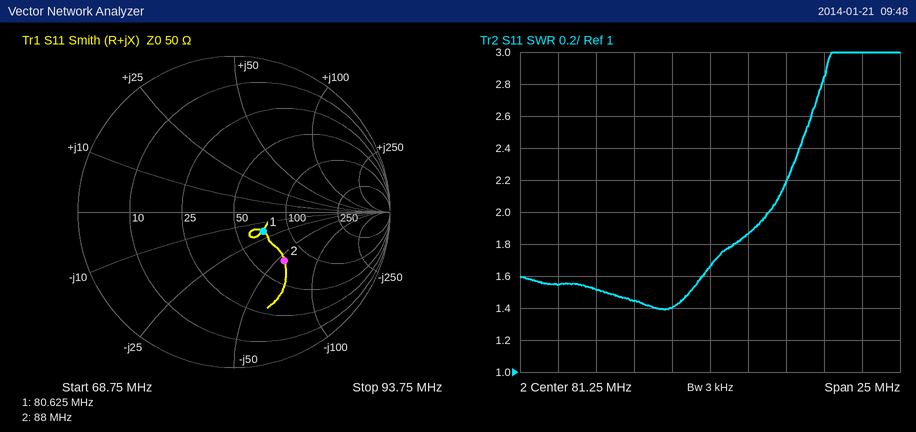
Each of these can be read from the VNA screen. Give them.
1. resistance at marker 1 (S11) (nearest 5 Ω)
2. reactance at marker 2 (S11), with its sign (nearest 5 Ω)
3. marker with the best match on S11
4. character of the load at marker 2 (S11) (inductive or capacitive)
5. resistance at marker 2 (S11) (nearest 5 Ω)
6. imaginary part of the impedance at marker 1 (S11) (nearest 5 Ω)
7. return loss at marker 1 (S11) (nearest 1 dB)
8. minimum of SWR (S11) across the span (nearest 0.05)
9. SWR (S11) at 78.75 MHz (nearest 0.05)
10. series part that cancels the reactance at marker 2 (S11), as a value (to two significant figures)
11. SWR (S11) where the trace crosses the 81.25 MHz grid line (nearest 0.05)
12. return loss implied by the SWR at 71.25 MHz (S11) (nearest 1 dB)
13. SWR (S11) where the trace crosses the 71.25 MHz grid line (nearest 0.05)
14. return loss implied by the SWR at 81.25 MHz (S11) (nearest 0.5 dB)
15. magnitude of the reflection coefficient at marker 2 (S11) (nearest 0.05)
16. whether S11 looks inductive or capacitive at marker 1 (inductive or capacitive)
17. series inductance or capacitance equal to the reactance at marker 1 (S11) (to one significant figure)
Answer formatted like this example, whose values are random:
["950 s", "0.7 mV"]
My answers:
["70 Ω", "-55 Ω", "marker 1", "capacitive", "70 Ω", "-20 Ω", "13 dB", "1.40", "1.40", "100 nH", "1.65", "13 dB", "1.55", "12.0 dB", "0.45", "capacitive", "100 pF"]
